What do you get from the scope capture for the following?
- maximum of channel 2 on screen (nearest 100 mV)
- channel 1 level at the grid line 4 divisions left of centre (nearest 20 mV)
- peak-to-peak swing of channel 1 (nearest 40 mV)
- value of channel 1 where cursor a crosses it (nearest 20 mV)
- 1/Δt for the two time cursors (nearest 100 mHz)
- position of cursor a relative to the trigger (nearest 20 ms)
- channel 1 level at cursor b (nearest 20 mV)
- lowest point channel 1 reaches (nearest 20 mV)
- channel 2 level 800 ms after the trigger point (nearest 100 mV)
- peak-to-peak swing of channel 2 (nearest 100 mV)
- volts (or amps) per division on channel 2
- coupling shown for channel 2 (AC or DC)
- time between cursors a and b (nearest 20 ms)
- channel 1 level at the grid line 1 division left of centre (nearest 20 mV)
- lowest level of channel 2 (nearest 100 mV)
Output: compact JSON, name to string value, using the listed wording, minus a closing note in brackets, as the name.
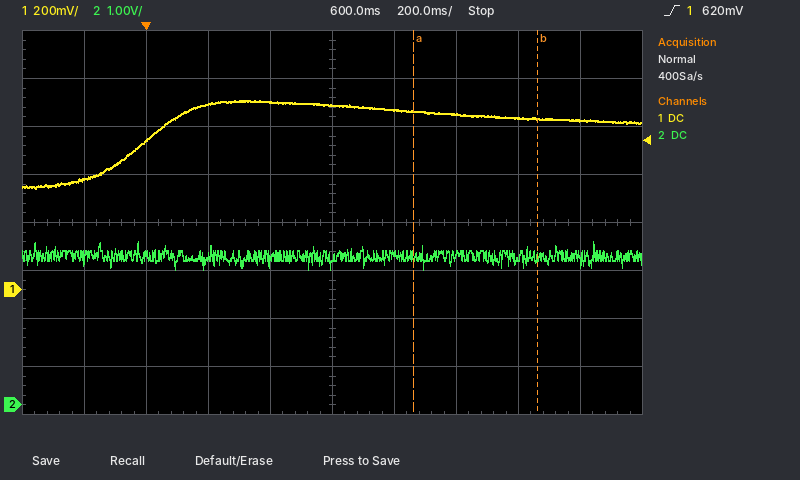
{"maximum of channel 2 on screen": "3.4 V", "channel 1 level at the grid line 4 divisions left of centre": "460 mV", "peak-to-peak swing of channel 1": "360 mV", "value of channel 1 where cursor a crosses it": "740 mV", "1/Δt for the two time cursors": "2.5 Hz", "position of cursor a relative to the trigger": "+860 ms", "channel 1 level at cursor b": "720 mV", "lowest point channel 1 reaches": "420 mV", "channel 2 level 800 ms after the trigger point": "3.1 V", "peak-to-peak swing of channel 2": "600 mV", "volts (or amps) per division on channel 2": "1 V", "coupling shown for channel 2": "DC", "time between cursors a and b": "400 ms", "channel 1 level at the grid line 1 division left of centre": "780 mV", "lowest level of channel 2": "2.8 V"}
